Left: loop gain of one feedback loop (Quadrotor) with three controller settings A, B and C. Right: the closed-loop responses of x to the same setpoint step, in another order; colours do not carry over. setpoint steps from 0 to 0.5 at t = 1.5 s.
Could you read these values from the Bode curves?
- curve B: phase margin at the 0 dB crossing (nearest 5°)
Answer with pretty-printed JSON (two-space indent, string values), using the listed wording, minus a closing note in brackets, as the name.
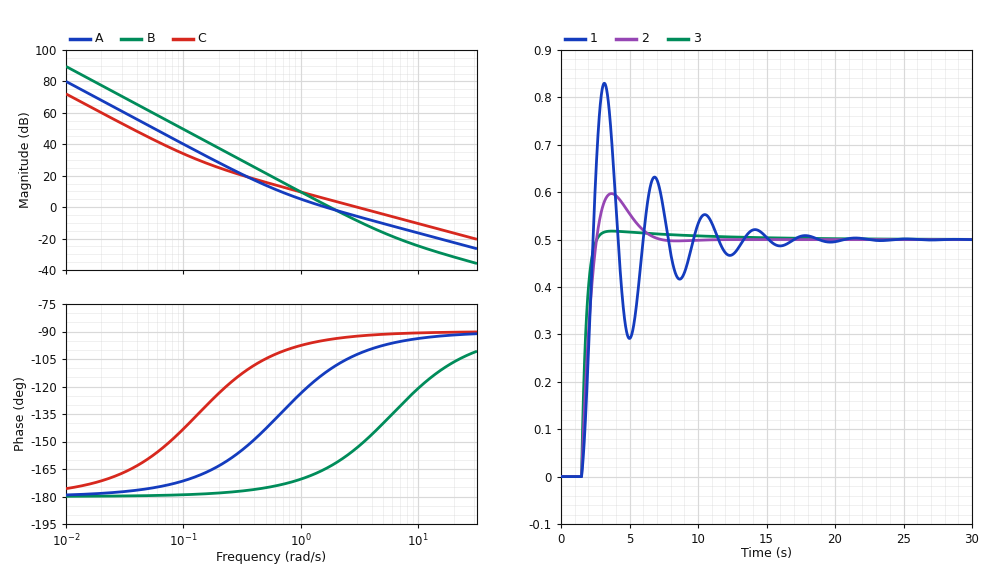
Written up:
{
  "curve B: phase margin at the 0 dB crossing": "15°"
}
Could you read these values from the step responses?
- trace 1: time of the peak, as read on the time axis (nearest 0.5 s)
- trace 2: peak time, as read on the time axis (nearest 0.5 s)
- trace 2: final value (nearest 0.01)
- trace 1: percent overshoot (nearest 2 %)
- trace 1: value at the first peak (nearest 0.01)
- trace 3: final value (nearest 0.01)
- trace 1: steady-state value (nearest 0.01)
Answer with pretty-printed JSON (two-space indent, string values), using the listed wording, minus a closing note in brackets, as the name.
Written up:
{
  "trace 1: time of the peak, as read on the time axis": "3.0 s",
  "trace 2: peak time, as read on the time axis": "3.5 s",
  "trace 2: final value": "0.50",
  "trace 1: percent overshoot": "66 %",
  "trace 1: value at the first peak": "0.83",
  "trace 3: final value": "0.50",
  "trace 1: steady-state value": "0.50"
}
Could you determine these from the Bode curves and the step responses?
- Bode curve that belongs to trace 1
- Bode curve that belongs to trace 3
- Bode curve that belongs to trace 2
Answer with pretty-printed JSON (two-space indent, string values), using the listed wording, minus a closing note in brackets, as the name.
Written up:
{
  "Bode curve that belongs to trace 1": "B",
  "Bode curve that belongs to trace 3": "C",
  "Bode curve that belongs to trace 2": "A"
}
